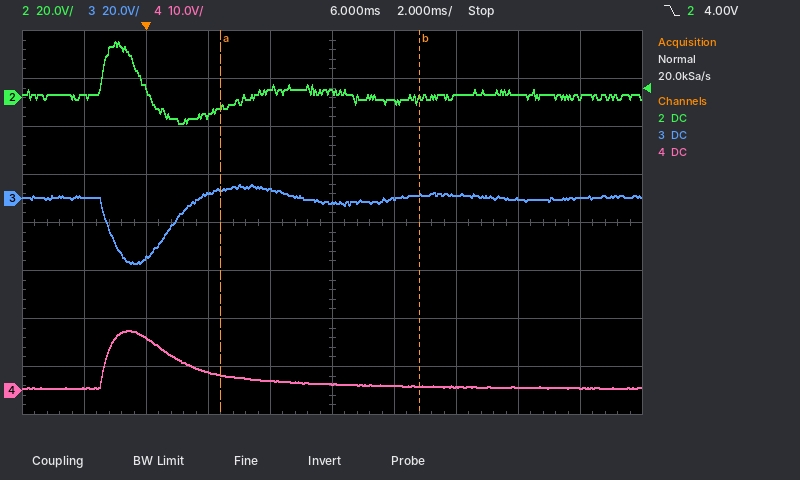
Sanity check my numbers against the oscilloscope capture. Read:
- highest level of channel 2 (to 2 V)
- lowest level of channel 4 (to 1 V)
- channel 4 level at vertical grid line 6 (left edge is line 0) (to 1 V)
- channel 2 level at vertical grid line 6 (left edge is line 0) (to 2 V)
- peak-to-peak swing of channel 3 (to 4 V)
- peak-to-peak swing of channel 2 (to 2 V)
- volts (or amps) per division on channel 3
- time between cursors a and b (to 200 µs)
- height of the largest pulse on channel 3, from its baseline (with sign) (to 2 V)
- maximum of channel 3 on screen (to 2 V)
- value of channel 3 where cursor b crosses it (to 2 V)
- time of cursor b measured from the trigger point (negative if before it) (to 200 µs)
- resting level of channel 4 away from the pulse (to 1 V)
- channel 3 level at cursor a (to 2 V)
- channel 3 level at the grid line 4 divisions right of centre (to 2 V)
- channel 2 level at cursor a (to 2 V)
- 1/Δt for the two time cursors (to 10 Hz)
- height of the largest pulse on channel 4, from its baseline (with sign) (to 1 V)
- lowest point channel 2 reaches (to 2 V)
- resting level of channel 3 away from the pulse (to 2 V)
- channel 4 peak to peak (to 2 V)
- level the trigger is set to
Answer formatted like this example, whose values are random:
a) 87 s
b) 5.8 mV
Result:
a) 24 V
b) 0 V
c) 1 V
d) -2 V
e) 32 V
f) 34 V
g) 20 V
h) 6.4 ms
i) -28 V
j) 6 V
k) 2 V
l) +8.8 ms
m) 1 V
n) 4 V
o) 0 V
p) -4 V
q) 160 Hz
r) +12 V
s) -10 V
t) 0 V
u) 12 V
v) 4.00 V
